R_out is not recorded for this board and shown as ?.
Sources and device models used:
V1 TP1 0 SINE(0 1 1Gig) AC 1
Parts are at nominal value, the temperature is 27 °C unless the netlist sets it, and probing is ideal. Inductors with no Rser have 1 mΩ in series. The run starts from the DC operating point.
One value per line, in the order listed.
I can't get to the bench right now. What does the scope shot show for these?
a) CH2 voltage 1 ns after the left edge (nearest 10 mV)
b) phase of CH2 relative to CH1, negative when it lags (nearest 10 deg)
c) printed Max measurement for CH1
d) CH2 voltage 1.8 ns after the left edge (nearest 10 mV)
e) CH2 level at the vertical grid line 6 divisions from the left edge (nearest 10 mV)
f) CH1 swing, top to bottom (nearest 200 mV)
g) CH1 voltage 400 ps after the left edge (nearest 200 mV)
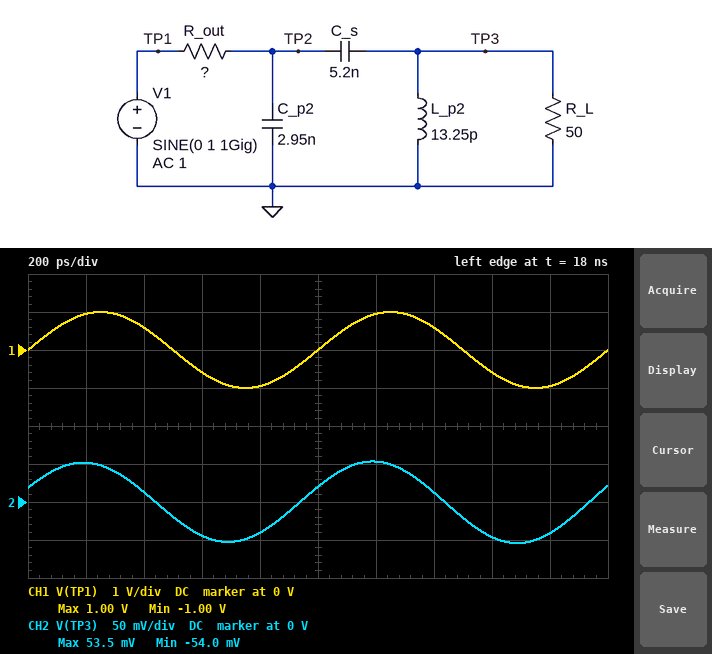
20 mV
20 deg
1.00 V
-40 mV
50 mV
2.0 V
600 mV
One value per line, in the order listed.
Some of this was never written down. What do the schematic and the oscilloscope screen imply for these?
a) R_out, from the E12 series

39 Ω
